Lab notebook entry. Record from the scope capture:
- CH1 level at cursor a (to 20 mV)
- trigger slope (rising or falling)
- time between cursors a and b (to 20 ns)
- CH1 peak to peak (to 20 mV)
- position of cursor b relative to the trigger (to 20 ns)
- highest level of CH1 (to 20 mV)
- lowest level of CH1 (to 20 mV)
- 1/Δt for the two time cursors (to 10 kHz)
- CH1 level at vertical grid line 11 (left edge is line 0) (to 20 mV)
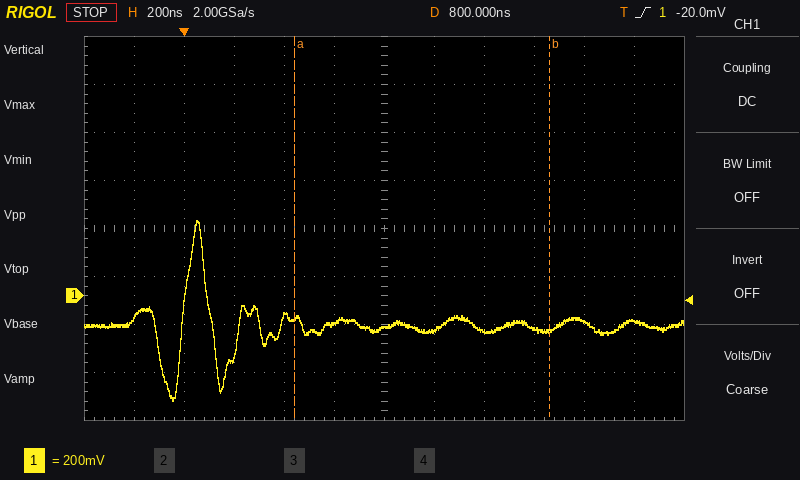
-100 mV
rising
1.02 µs
760 mV
+1.46 µs
320 mV
-440 mV
980 kHz
-100 mV
